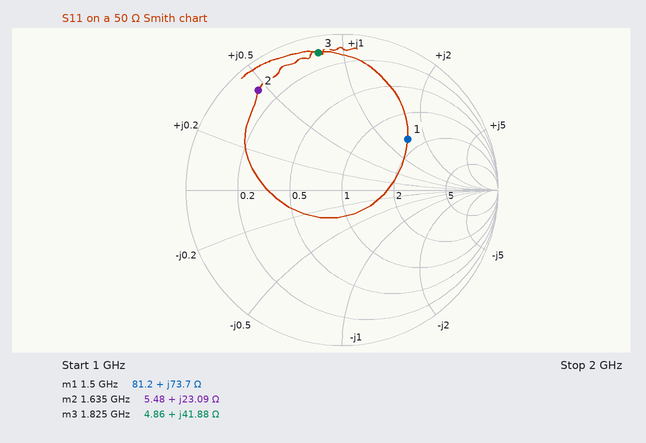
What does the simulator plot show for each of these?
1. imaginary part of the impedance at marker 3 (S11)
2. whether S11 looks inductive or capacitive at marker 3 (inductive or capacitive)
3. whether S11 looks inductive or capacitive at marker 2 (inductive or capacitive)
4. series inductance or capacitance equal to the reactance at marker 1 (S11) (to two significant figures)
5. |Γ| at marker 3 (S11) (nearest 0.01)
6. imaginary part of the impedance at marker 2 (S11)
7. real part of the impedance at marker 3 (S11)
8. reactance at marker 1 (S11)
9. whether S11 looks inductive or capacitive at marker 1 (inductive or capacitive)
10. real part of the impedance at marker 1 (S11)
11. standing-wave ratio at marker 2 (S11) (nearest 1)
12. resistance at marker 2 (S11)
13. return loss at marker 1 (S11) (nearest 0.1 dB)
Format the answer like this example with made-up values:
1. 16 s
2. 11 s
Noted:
1. +41.88 Ω
2. inductive
3. inductive
4. 7.8 nH
5. 0.89
6. +23.09 Ω
7. 4.86 Ω
8. +73.7 Ω
9. inductive
10. 81.2 Ω
11. 11
12. 5.48 Ω
13. 5.5 dB
